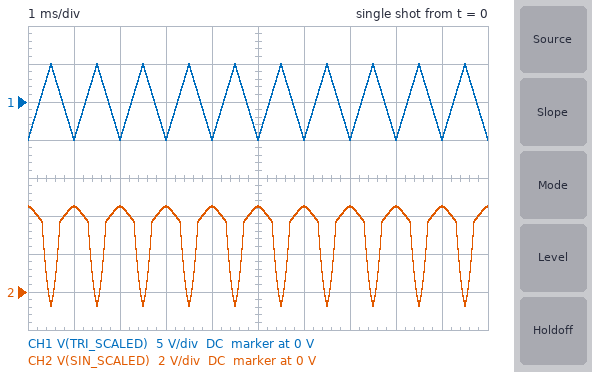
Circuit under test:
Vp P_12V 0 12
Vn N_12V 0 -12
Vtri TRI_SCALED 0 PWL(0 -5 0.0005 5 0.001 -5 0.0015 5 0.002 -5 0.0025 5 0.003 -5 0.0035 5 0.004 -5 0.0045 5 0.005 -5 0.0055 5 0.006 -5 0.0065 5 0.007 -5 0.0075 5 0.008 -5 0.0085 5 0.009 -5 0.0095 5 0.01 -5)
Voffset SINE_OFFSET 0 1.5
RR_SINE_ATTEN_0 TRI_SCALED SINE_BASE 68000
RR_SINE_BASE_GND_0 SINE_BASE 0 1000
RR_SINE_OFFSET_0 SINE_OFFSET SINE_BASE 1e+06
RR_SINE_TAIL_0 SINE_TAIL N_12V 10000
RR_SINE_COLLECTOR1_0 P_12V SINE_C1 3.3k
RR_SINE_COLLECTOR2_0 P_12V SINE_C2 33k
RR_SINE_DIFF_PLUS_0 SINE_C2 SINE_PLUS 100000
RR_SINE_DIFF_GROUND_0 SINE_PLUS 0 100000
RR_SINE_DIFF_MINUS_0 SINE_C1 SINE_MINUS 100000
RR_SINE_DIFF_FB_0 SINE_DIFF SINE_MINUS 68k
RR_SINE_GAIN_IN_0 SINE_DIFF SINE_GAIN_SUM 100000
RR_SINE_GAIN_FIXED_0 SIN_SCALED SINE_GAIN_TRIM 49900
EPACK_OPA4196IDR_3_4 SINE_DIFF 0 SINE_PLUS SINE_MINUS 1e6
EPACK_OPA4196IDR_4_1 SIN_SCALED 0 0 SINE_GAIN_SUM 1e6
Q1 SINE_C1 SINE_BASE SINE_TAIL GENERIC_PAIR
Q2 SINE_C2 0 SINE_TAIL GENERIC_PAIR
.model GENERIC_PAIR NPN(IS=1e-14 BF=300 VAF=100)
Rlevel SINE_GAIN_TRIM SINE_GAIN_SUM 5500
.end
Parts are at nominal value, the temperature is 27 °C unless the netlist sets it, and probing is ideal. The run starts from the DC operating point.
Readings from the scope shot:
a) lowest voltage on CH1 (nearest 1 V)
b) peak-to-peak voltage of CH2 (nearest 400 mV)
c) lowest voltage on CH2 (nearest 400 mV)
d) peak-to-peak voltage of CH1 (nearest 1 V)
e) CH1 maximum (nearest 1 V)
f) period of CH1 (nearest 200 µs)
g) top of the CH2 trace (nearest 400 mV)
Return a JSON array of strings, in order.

["-5 V", "5.2 V", "-800 mV", "10 V", "5 V", "1.0 ms", "4.4 V"]
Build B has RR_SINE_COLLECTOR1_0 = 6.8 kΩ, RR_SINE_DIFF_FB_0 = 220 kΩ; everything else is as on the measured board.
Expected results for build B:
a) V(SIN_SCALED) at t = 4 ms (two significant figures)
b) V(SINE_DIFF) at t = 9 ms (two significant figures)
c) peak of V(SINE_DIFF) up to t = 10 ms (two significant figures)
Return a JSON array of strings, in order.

["13 V", "-24 V", "2.8 V"]
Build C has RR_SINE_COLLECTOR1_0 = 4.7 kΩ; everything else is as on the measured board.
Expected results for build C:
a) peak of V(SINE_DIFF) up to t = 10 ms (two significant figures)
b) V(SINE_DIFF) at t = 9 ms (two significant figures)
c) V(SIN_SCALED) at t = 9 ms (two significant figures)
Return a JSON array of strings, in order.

["2.3 V", "-8.0 V", "4.4 V"]
